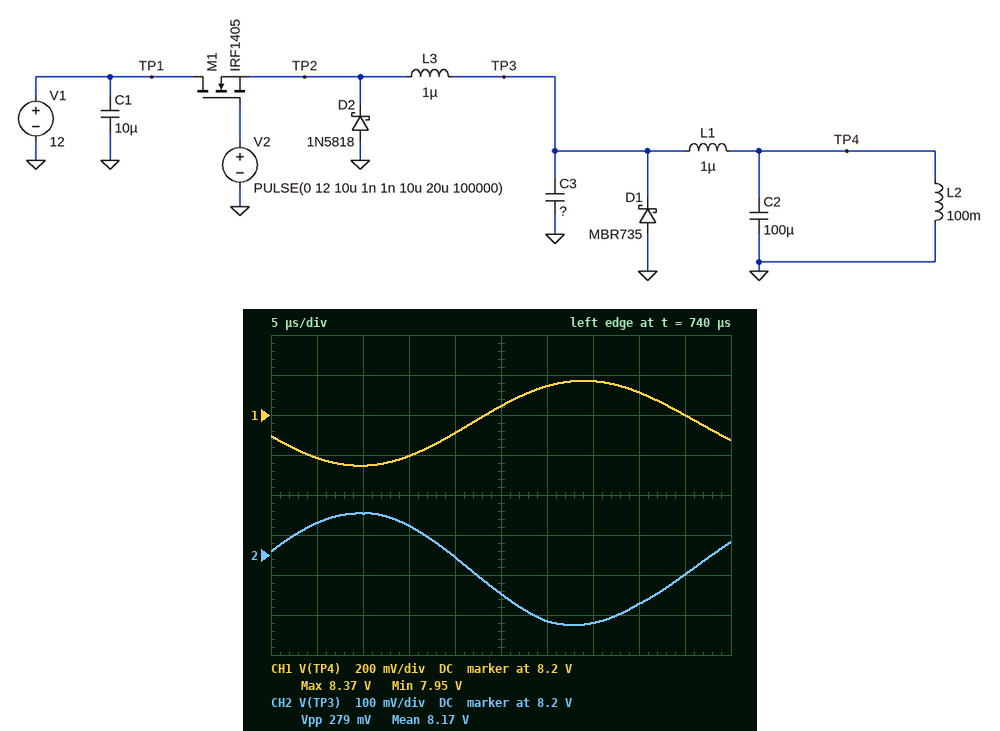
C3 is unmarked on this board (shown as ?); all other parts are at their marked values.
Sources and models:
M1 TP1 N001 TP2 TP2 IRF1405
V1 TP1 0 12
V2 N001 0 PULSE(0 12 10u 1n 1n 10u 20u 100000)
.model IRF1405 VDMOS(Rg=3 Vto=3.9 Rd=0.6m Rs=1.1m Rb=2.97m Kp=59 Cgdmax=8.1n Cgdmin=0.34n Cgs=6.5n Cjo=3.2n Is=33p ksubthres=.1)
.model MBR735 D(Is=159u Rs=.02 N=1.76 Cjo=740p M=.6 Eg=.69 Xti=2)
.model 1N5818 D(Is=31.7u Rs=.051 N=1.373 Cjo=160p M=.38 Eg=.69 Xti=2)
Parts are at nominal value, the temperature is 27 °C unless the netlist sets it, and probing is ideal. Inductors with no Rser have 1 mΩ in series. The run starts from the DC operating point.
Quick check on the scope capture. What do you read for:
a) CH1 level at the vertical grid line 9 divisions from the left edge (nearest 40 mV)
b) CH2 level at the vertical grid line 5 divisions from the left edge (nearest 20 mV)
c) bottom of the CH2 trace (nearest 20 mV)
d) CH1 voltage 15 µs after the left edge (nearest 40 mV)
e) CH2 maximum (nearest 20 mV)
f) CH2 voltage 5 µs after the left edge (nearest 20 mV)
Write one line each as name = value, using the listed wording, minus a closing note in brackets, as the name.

CH1 level at the vertical grid line 9 divisions from the left edge = 8.20 V
CH2 level at the vertical grid line 5 divisions from the left edge = 8.10 V
bottom of the CH2 trace = 8.02 V
CH1 voltage 15 µs after the left edge = 8.00 V
CH2 maximum = 8.30 V
CH2 voltage 5 µs after the left edge = 8.28 V
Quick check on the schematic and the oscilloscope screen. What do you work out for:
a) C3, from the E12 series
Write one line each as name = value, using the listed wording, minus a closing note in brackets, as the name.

C3, from the E12 series = 150 µF
